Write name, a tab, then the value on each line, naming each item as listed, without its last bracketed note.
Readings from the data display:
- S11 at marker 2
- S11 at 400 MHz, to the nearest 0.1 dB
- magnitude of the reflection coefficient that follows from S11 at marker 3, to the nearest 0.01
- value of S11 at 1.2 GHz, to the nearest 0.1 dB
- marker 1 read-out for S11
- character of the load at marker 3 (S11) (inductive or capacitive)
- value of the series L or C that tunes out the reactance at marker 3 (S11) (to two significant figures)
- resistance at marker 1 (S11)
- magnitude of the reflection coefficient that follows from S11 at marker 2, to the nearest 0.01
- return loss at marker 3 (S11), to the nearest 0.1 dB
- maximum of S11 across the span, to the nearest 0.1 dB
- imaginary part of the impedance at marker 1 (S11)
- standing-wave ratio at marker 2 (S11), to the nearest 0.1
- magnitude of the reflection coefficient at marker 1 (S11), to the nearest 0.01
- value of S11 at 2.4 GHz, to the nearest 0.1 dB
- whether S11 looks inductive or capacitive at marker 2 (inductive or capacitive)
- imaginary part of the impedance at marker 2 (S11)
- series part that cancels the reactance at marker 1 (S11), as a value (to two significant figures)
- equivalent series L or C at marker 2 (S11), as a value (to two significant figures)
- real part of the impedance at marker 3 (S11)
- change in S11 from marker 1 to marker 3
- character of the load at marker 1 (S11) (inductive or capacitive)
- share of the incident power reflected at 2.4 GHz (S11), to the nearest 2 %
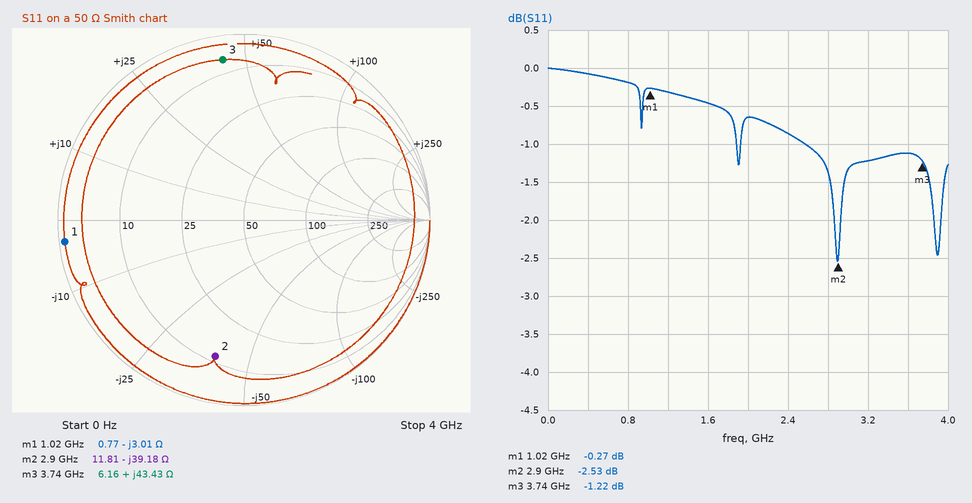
S11 at marker 2	-2.53 dB
S11 at 400 MHz, to the nearest 0.1 dB	-0.1 dB
magnitude of the reflection coefficient that follows from S11 at marker 3, to the nearest 0.01	0.87
value of S11 at 1.2 GHz, to the nearest 0.1 dB	-0.3 dB
marker 1 read-out for S11	-0.27 dB
character of the load at marker 3 (S11)	inductive
value of the series L or C that tunes out the reactance at marker 3 (S11)	980 fF
resistance at marker 1	0.77 Ω
magnitude of the reflection coefficient that follows from S11 at marker 2, to the nearest 0.01	0.75
return loss at marker 3 (S11), to the nearest 0.1 dB	1.2 dB
maximum of S11 across the span, to the nearest 0.1 dB	0.0 dB
imaginary part of the impedance at marker 1	-3.01 Ω
standing-wave ratio at marker 2 (S11), to the nearest 0.1	6.9
magnitude of the reflection coefficient at marker 1 (S11), to the nearest 0.01	0.97
value of S11 at 2.4 GHz, to the nearest 0.1 dB	-0.9 dB
whether S11 looks inductive or capacitive at marker 2	capacitive
imaginary part of the impedance at marker 2	-39.18 Ω
series part that cancels the reactance at marker 1 (S11), as a value	470 pH
equivalent series L or C at marker 2 (S11), as a value	1.4 pF
real part of the impedance at marker 3	6.16 Ω
change in S11 from marker 1 to marker 3	-0.95 dB
character of the load at marker 1 (S11)	capacitive
share of the incident power reflected at 2.4 GHz (S11), to the nearest 2 %	82 %
